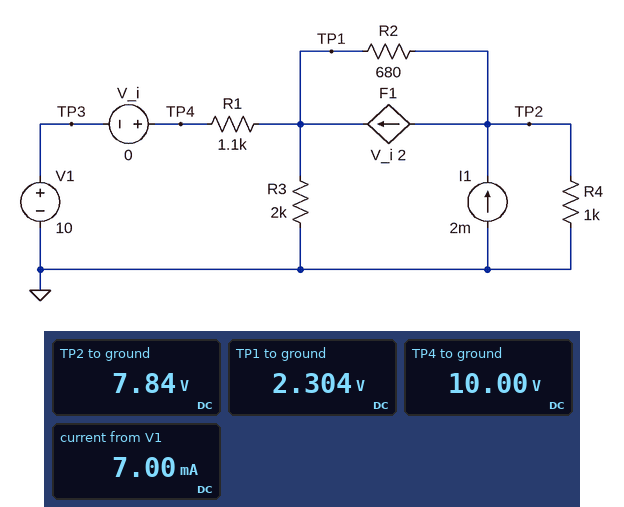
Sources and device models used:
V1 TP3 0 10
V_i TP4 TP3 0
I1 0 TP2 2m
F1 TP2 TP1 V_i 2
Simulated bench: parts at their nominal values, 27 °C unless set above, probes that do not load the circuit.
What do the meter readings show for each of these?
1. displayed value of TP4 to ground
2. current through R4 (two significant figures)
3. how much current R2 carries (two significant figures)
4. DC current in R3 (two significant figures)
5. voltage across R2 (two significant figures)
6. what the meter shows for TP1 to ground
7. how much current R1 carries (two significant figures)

10.00 V
7.8 mA
8.1 mA
1.2 mA
5.5 V
2.304 V
7.0 mA
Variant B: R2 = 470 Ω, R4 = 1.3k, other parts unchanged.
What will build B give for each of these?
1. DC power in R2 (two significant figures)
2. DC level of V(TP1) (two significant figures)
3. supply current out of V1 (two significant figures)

27 mW
3.8 V
5.6 mA
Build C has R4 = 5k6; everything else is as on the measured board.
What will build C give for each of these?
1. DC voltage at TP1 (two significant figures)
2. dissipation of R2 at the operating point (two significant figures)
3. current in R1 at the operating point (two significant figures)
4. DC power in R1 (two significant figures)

6.5 V
28 mW
3.2 mA
11 mW
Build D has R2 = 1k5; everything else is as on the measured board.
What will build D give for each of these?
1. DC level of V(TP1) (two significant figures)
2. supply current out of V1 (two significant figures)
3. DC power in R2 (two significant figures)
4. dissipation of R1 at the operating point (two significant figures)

-1.4 V
10 mA
140 mW
120 mW
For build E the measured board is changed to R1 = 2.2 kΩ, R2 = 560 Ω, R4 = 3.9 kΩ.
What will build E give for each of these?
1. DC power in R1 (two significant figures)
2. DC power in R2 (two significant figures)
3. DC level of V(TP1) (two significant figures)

12 mW
13 mW
4.8 V
